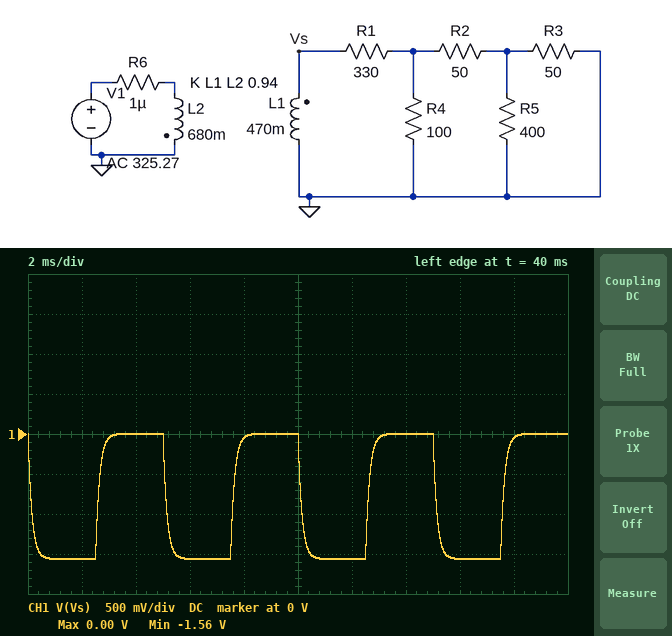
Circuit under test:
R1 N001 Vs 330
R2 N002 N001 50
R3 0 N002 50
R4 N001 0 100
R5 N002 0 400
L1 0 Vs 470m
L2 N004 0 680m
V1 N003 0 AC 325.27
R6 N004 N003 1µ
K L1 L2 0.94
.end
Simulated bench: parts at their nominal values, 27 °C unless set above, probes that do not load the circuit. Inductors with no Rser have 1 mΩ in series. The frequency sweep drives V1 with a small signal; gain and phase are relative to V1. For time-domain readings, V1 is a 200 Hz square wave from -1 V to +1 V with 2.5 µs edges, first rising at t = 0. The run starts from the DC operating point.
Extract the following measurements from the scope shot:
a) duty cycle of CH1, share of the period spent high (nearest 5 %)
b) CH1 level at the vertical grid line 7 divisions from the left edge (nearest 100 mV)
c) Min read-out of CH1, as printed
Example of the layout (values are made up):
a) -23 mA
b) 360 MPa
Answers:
a) 50 %
b) 0 V
c) -1.56 V
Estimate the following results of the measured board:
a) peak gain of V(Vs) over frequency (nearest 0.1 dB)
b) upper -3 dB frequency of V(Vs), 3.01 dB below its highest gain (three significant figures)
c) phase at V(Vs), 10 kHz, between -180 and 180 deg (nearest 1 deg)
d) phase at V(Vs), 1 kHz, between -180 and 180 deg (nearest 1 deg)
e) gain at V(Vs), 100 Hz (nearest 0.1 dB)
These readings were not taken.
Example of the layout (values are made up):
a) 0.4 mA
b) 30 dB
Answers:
a) -2.1 dB
b) 1.10 kHz
c) 96 deg
d) 138 deg
e) -2.2 dB
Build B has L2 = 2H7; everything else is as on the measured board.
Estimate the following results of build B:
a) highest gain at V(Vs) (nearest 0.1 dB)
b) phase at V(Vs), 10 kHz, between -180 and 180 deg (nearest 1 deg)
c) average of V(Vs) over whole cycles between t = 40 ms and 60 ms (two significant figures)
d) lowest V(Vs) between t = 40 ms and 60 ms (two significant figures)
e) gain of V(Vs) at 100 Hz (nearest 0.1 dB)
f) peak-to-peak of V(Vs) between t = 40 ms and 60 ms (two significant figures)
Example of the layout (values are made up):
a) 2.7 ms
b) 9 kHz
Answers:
a) -8.1 dB
b) 96 deg
c) -390 mV
d) -780 mV
e) -8.2 dB
f) 780 mV
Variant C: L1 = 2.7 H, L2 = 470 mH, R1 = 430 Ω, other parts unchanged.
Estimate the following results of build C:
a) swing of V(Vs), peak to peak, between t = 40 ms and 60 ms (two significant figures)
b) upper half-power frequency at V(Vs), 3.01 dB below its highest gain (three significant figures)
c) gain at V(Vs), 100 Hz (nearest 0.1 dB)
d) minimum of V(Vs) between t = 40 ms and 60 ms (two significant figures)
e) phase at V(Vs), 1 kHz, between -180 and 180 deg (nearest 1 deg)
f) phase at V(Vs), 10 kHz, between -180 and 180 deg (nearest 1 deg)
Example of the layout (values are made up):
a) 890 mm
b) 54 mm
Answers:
a) 4.3 V
b) 242 Hz
c) 6.4 dB
d) -4.4 V
e) 104 deg
f) 91 deg
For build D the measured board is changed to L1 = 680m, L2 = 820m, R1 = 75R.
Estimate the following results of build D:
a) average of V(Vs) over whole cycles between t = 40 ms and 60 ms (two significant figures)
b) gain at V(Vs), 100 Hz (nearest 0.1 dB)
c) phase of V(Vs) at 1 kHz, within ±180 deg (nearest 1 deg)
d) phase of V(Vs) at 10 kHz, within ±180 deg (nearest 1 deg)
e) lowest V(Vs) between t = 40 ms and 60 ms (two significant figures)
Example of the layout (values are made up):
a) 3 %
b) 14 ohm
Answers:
a) -860 mV
b) -2.0 dB
c) 104 deg
d) 91 deg
e) -1.7 V
